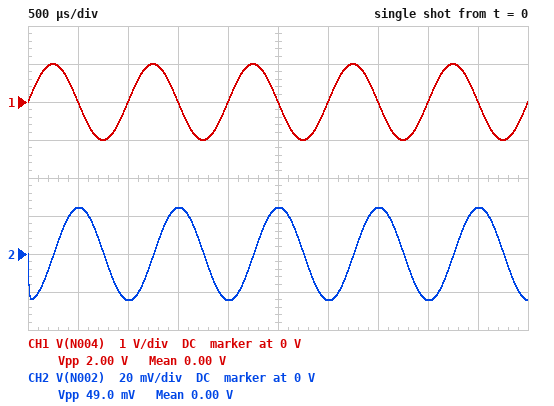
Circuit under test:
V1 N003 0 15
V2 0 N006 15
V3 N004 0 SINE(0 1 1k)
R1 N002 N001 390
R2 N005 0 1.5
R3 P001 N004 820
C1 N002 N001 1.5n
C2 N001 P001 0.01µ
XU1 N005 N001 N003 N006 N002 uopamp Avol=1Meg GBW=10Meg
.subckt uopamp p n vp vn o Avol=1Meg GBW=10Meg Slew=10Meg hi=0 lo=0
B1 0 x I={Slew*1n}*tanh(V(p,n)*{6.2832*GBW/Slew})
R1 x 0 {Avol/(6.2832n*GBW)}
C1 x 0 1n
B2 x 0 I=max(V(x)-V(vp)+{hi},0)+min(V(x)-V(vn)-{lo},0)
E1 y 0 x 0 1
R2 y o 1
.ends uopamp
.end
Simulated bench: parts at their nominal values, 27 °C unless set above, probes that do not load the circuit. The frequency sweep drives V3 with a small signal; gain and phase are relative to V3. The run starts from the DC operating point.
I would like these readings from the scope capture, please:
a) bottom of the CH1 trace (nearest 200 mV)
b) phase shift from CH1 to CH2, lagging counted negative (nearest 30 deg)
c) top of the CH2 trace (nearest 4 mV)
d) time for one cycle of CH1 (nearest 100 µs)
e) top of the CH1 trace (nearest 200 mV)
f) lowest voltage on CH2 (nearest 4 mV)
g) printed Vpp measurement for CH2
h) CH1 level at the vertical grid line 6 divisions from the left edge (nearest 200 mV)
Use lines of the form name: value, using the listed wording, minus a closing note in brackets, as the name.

bottom of the CH1 trace: -1.0 V
phase shift from CH1 to CH2, lagging counted negative: -90 deg
top of the CH2 trace: 24 mV
time for one cycle of CH1: 1.0 ms
top of the CH1 trace: 1.0 V
lowest voltage on CH2: -24 mV
printed Vpp measurement for CH2: 49.0 mV
CH1 level at the vertical grid line 6 divisions from the left edge: 0 V
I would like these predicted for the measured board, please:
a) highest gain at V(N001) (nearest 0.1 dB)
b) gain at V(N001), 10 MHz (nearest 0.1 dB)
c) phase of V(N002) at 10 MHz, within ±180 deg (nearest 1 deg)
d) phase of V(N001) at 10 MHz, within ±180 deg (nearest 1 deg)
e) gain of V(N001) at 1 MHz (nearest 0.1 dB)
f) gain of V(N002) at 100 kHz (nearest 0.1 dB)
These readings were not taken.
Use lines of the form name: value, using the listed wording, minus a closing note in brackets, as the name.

highest gain at V(N001): -38.1 dB
gain at V(N001), 10 MHz: -40.8 dB
phase of V(N002) at 10 MHz, within ±180 deg: 47 deg
phase of V(N001) at 10 MHz, within ±180 deg: -38 deg
gain of V(N001) at 1 MHz: -38.2 dB
gain of V(N002) at 100 kHz: -7.2 dB
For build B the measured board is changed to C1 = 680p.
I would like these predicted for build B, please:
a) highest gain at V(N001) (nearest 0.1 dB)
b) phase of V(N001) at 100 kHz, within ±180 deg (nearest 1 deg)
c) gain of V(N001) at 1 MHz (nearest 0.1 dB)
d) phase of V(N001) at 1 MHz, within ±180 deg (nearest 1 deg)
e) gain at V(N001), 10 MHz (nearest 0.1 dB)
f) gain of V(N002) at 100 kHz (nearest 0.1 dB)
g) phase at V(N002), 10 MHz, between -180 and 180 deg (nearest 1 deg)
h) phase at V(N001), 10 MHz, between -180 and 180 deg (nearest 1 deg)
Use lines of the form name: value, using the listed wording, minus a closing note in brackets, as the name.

highest gain at V(N001): -31.6 dB
phase of V(N001) at 100 kHz, within ±180 deg: 91 deg
gain of V(N001) at 1 MHz: -32.4 dB
phase of V(N001) at 1 MHz, within ±180 deg: 26 deg
gain at V(N001), 10 MHz: -34.0 dB
gain of V(N002) at 100 kHz: -6.7 dB
phase at V(N002), 10 MHz, between -180 and 180 deg: 49 deg
phase at V(N001), 10 MHz, between -180 and 180 deg: -38 deg
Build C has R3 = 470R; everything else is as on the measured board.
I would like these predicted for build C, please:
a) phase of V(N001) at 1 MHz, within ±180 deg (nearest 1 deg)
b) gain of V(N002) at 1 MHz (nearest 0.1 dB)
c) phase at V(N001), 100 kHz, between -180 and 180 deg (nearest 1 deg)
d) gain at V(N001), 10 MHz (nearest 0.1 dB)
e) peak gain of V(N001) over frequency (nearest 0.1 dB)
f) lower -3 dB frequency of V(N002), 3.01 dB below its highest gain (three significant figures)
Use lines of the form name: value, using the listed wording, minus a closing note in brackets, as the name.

phase of V(N001) at 1 MHz, within ±180 deg: 12 deg
gain of V(N002) at 1 MHz: -13.5 dB
phase at V(N001), 100 kHz, between -180 and 180 deg: 88 deg
gain at V(N001), 10 MHz: -36.0 dB
peak gain of V(N001) over frequency: -33.3 dB
lower -3 dB frequency of V(N002), 3.01 dB below its highest gain: 27.6 kHz
